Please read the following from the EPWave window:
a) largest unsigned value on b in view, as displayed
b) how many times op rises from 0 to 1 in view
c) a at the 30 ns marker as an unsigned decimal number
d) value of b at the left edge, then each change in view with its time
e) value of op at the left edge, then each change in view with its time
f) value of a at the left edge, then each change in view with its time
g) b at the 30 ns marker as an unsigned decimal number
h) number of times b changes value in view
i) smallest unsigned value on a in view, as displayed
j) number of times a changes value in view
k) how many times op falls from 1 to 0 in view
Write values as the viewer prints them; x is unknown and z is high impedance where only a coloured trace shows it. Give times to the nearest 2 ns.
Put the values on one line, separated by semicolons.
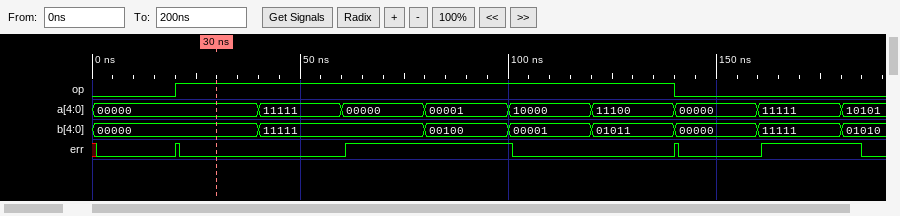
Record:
11111; 1; 0; 00000, 11111 at 40 ns, 00100 at 80 ns, 00001 at 100 ns, 01011 at 120 ns, 00000 at 140 ns, 11111 at 160 ns, 01010 at 180 ns; 0, 1 at 20 ns, 0 at 140 ns; 00000, 11111 at 40 ns, 00000 at 60 ns, 00001 at 80 ns, 10000 at 100 ns, 11100 at 120 ns, 00000 at 140 ns, 11111 at 160 ns, 10101 at 180 ns; 0; 7; 00000; 8; 1
